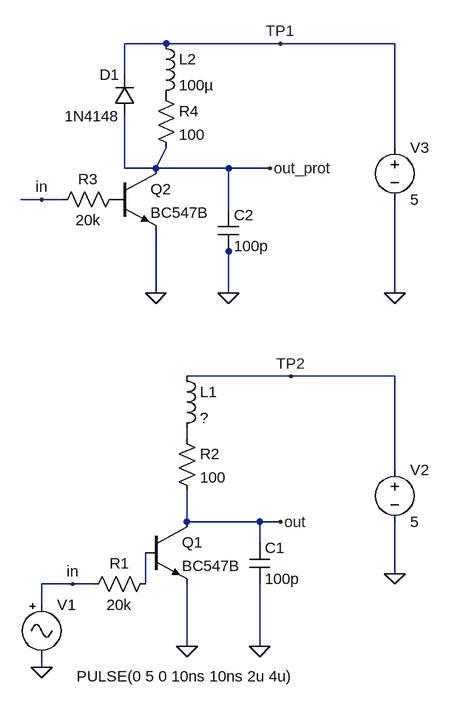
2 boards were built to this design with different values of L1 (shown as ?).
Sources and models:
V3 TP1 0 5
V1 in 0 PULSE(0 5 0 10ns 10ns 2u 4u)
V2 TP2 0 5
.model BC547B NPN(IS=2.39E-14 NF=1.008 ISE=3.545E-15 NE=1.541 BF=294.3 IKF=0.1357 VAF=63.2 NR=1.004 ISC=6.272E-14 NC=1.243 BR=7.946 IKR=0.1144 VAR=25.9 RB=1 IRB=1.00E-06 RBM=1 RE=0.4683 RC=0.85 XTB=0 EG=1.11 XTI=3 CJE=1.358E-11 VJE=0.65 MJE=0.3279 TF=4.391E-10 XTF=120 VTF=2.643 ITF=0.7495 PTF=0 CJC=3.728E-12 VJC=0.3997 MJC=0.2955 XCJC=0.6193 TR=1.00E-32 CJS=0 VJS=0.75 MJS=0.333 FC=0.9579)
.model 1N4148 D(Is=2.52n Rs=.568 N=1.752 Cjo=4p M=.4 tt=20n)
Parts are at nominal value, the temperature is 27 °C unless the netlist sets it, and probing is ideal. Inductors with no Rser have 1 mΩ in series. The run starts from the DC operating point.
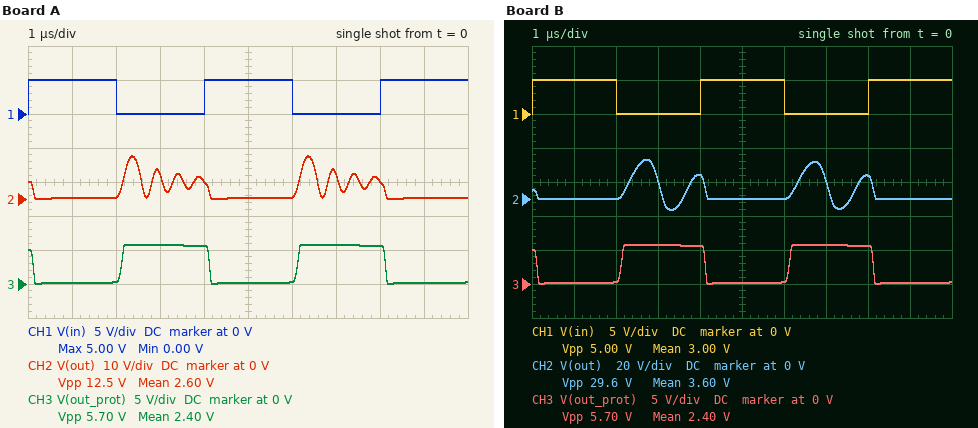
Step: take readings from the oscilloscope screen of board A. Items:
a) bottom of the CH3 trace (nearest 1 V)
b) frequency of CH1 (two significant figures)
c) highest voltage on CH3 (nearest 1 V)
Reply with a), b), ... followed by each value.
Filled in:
a) 0 V
b) 250 kHz
c) 6 V
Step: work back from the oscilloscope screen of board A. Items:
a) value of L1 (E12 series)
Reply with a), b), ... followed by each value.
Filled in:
a) 56 µH
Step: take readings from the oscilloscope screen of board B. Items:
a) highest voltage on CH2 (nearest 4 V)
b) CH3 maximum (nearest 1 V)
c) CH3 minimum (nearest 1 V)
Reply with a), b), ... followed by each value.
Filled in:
a) 24 V
b) 6 V
c) 0 V
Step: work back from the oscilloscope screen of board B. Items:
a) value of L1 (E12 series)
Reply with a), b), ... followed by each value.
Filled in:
a) 330 µH
